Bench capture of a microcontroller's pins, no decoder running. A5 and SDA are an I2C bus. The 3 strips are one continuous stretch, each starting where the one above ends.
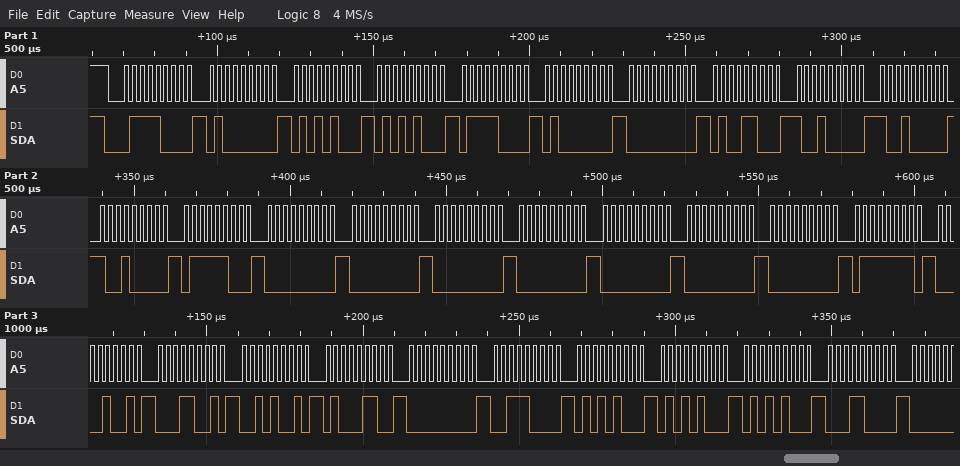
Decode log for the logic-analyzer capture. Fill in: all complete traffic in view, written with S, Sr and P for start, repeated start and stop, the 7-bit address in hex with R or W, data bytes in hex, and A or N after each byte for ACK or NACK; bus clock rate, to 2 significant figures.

S 3CW A 40 A 54 A 54 A 78 A 40 A 00 A 4C A 90 A 90 A 90 A 7C A 00 A 00 A 00 A 00 A 00 A 00 A 00 A 7F A 09 A 19 A 29 A 46 A 00 A 38 A 54 A 54 A 54 A 18 A
400 kHz
